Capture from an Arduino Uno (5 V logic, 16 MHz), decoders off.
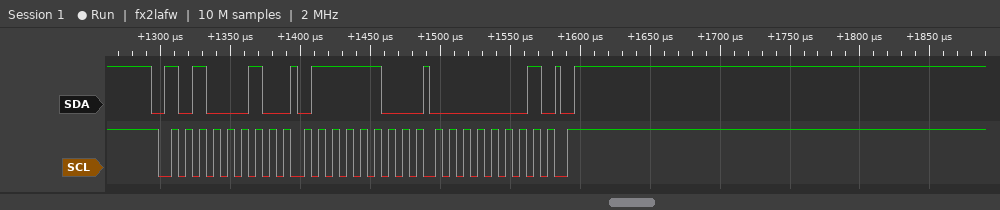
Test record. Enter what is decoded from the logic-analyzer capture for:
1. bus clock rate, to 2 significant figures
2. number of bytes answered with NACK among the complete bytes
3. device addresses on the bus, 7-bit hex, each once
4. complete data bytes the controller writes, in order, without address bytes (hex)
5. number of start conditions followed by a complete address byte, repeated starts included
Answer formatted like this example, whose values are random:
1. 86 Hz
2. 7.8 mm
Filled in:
1. 100 kHz
2. 0
3. 0x51
4. 7C 01
5. 1
